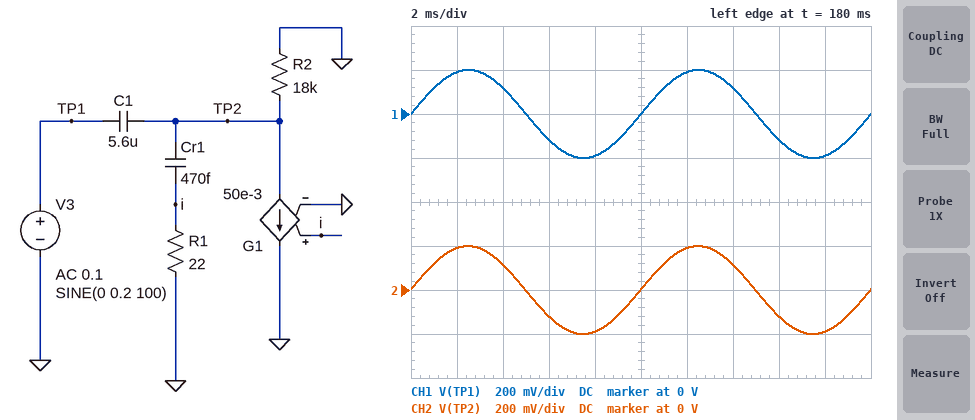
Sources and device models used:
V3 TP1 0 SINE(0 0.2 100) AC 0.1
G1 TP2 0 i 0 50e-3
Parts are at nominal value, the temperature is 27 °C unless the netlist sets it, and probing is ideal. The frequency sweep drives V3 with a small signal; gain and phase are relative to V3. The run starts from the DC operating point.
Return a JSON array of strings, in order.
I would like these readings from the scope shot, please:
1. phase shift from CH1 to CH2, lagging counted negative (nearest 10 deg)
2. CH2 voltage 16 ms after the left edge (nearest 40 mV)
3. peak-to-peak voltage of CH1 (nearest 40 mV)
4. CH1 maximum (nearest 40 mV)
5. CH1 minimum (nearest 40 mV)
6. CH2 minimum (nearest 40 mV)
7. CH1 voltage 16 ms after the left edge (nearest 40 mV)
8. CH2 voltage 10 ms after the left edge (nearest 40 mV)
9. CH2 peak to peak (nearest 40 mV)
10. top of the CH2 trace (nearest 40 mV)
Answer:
["0 deg", "-120 mV", "400 mV", "200 mV", "-200 mV", "-200 mV", "-120 mV", "0 V", "400 mV", "200 mV"]
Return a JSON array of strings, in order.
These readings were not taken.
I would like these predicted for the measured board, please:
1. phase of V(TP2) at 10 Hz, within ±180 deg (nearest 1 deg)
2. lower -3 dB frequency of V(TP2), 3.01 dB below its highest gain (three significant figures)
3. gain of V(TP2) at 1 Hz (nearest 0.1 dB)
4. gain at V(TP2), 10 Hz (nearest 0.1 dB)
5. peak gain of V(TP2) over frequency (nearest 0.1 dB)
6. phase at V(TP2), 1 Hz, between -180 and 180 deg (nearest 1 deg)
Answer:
["9 deg", "1.58 Hz", "-5.4 dB", "-0.1 dB", "0 dB", "58 deg"]
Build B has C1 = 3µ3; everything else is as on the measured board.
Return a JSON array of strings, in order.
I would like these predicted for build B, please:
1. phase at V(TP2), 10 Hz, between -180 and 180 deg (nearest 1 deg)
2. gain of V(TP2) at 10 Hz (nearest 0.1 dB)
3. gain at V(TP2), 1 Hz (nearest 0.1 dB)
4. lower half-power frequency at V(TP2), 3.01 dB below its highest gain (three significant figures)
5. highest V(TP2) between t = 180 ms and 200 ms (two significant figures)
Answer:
["15 deg", "-0.3 dB", "-9.1 dB", "2.68 Hz", "200 mV"]
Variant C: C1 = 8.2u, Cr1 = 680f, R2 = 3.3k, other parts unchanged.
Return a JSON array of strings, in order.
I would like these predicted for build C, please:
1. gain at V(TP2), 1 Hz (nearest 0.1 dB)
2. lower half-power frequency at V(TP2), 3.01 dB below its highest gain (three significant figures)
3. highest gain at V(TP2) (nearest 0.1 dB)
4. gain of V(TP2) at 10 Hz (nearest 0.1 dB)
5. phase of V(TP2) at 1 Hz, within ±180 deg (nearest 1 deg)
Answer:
["-15.5 dB", "5.88 Hz", "0 dB", "-1.3 dB", "80 deg"]
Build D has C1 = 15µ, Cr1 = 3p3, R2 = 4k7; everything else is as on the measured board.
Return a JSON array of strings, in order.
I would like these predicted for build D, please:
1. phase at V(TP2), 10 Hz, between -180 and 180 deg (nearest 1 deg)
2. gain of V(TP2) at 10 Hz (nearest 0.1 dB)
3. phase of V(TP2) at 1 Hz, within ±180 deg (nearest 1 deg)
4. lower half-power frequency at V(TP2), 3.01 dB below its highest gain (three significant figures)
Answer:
["13 deg", "-0.2 dB", "66 deg", "2.26 Hz"]
